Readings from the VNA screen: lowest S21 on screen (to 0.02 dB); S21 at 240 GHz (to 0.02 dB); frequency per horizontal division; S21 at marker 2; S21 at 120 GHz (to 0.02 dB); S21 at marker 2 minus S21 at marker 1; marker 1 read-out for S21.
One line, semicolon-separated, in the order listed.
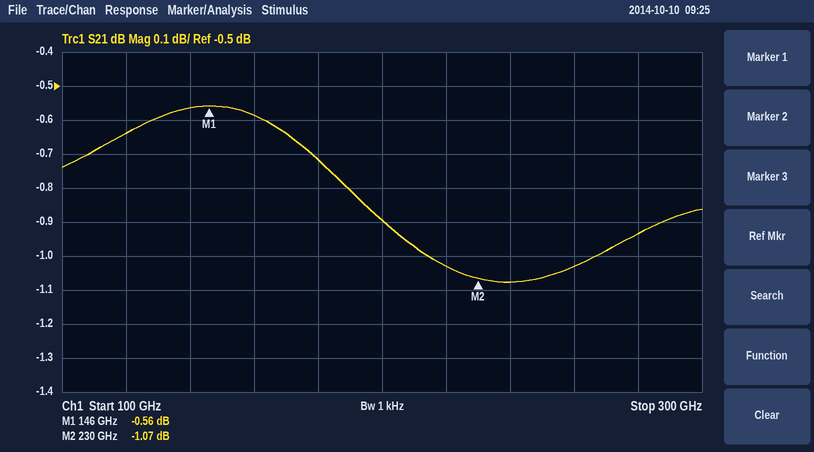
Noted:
-1.08 dB; -1.08 dB; 20 GHz; -1.07 dB; -0.64 dB; -0.51 dB; -0.56 dB
